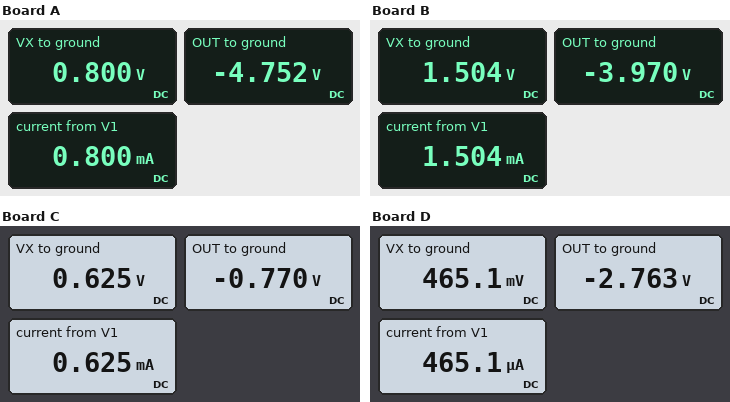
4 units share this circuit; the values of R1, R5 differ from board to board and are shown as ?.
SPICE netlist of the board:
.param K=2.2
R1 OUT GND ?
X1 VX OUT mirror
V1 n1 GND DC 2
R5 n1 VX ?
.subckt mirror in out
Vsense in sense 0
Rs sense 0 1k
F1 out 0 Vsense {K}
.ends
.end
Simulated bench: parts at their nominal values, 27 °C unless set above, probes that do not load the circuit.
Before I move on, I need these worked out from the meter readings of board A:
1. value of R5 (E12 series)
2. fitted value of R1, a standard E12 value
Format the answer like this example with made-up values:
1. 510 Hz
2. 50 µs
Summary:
1. 1.5 kΩ
2. 2.7 kΩ
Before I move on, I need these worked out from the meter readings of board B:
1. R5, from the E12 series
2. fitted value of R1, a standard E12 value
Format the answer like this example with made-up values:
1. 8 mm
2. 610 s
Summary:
1. 330 Ω
2. 1.2 kΩ
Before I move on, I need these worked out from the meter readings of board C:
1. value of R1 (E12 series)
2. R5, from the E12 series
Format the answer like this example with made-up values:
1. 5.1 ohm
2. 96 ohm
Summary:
1. 560 Ω
2. 2.2 kΩ
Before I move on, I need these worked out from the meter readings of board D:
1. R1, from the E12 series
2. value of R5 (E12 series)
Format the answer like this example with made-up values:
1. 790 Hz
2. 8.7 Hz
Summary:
1. 2.7 kΩ
2. 3.3 kΩ
